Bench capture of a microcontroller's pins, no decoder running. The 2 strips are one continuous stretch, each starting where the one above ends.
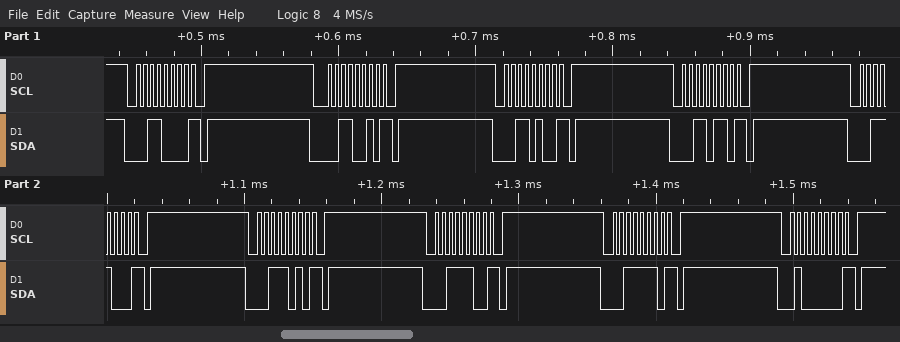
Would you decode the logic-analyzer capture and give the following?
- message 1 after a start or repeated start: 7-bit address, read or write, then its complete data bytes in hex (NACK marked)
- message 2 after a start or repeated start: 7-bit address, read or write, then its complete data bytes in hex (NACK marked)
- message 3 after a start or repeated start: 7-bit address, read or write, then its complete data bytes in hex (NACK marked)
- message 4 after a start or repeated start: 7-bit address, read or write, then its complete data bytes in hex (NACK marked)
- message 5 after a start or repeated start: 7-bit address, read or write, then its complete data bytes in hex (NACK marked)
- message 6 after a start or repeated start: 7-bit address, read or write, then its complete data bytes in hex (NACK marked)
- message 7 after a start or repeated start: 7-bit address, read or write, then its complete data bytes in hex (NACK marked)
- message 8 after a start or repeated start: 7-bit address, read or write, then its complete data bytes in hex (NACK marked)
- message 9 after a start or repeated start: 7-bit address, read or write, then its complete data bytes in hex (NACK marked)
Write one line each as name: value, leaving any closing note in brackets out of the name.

message 1 after a start or repeated start: 7-bit address, read or write, then its complete data bytes in hex: 0x18 write NACK
message 2 after a start or repeated start: 7-bit address, read or write, then its complete data bytes in hex: 0x19 write NACK
message 3 after a start or repeated start: 7-bit address, read or write, then its complete data bytes in hex: 0x1A write NACK
message 4 after a start or repeated start: 7-bit address, read or write, then its complete data bytes in hex: 0x1B write NACK
message 5 after a start or repeated start: 7-bit address, read or write, then its complete data bytes in hex: 0x1C write NACK
message 6 after a start or repeated start: 7-bit address, read or write, then its complete data bytes in hex: 0x1D write NACK
message 7 after a start or repeated start: 7-bit address, read or write, then its complete data bytes in hex: 0x1E write NACK
message 8 after a start or repeated start: 7-bit address, read or write, then its complete data bytes in hex: 0x1F write NACK
message 9 after a start or repeated start: 7-bit address, read or write, then its complete data bytes in hex: 0x20 write NACK
